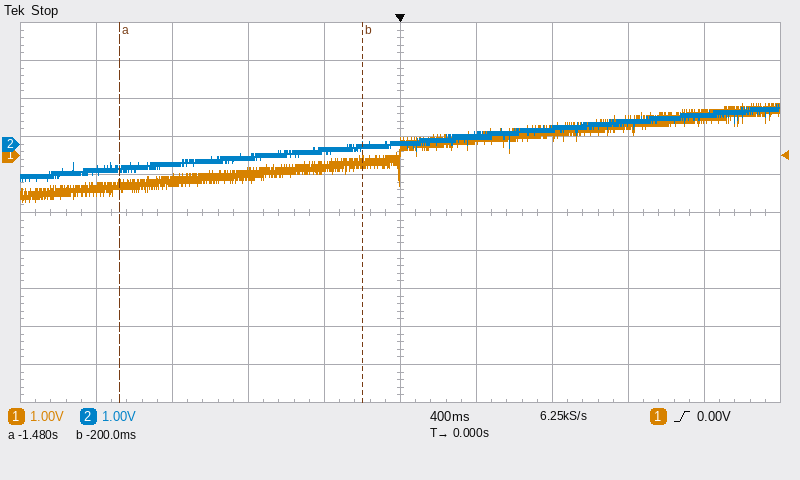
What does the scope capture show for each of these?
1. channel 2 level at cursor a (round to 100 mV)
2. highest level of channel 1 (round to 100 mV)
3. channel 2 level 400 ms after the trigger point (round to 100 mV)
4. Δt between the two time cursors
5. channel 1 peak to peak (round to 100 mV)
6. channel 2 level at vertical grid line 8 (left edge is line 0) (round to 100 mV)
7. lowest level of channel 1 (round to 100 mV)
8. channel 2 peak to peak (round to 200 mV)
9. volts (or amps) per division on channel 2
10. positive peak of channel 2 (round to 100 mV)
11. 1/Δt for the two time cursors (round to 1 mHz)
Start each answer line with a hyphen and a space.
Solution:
- -600 mV
- 1.4 V
- 200 mV
- 1.28 s
- 2.6 V
- 600 mV
- -1.2 V
- 2.0 V
- 1 V
- 1.0 V
- 781 mHz
